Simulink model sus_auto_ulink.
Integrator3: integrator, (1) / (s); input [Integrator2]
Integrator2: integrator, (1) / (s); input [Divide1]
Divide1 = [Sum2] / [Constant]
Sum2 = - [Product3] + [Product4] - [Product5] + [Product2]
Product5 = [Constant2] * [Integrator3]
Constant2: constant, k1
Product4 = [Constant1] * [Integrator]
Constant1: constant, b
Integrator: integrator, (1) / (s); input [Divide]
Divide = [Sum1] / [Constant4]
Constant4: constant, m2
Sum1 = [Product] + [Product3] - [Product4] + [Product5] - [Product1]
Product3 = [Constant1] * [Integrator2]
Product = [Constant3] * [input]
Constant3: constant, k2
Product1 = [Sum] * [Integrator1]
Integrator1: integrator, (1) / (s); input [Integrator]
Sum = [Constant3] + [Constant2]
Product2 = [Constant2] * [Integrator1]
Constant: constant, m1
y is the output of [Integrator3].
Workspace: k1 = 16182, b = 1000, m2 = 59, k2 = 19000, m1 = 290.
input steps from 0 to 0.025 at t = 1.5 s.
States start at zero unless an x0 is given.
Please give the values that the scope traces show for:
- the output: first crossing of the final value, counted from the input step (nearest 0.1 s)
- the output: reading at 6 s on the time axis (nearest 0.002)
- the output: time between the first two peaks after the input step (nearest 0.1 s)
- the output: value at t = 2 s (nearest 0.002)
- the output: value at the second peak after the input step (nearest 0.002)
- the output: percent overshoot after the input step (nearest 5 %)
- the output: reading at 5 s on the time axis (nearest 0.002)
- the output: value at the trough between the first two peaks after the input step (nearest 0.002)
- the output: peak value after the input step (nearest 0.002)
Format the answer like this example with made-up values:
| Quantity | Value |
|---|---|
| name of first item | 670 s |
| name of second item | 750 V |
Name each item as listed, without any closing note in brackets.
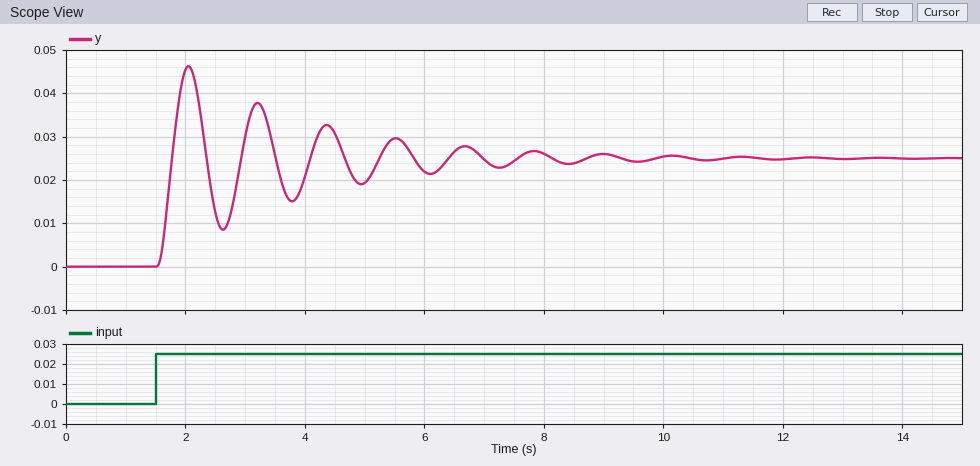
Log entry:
| Quantity | Value |
|---|---|
| the output: first crossing of the final value, counted from the input step | 0.3 s |
| the output: reading at 6 s on the time axis | 0.022 |
| the output: time between the first two peaks after the input step | 1.2 s |
| the output: value at t = 2 s | 0.046 |
| the output: value at the second peak after the input step | 0.038 |
| the output: percent overshoot after the input step | 85 % |
| the output: reading at 5 s on the time axis | 0.020 |
| the output: value at the trough between the first two peaks after the input step | 0.008 |
| the output: peak value after the input step | 0.046 |
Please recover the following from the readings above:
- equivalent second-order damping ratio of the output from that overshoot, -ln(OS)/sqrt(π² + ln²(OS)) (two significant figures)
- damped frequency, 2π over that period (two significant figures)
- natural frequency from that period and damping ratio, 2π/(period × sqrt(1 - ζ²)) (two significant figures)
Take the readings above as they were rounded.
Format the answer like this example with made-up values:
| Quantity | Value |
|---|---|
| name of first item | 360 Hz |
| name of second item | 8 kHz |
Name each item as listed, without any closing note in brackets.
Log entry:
| Quantity | Value |
|---|---|
| equivalent second-order damping ratio of the output from that overshoot, -ln(OS)/sqrt(π² + ln²(OS)) | 0.052 |
| damped frequency, 2π over that period | 5.2 rad/s |
| natural frequency from that period and damping ratio, 2π/(period × sqrt(1 - ζ²)) | 5.2 rad/s |
